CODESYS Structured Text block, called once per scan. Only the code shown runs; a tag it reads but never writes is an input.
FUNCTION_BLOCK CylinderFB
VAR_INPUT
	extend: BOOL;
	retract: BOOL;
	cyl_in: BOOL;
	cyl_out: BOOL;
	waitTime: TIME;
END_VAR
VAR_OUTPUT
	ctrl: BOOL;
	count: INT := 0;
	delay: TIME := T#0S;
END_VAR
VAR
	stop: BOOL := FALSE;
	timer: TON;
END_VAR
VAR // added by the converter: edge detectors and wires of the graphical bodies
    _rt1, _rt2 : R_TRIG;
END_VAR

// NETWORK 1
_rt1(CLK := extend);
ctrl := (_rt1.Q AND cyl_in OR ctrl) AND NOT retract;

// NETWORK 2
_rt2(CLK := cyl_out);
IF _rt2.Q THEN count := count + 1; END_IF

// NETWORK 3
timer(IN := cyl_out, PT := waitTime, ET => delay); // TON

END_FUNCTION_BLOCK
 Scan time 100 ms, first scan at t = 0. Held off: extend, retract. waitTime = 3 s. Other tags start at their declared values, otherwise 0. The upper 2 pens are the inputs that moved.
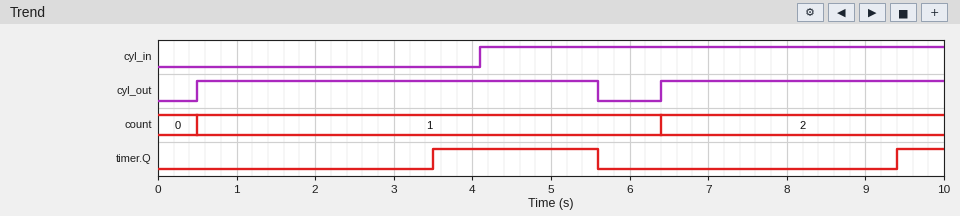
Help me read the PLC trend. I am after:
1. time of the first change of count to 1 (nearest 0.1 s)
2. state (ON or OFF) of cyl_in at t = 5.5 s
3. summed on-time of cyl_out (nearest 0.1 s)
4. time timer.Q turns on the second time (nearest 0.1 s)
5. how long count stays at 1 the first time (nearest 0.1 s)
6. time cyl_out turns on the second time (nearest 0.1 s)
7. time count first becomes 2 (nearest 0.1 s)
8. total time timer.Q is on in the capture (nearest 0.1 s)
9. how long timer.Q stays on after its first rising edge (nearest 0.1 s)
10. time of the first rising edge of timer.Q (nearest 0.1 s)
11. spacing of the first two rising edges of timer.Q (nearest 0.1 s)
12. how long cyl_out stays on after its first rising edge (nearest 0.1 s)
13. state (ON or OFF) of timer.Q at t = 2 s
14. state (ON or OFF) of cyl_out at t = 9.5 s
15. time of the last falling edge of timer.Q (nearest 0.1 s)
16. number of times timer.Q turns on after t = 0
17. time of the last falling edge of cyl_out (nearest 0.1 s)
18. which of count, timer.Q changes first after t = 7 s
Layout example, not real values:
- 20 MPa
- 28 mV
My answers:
- 0.5 s
- ON
- 8.7 s
- 9.4 s
- 5.9 s
- 6.4 s
- 6.4 s
- 2.7 s
- 2.1 s
- 3.5 s
- 5.9 s
- 5.1 s
- OFF
- ON
- 5.6 s
- 2
- 5.6 s
- timer.Q
